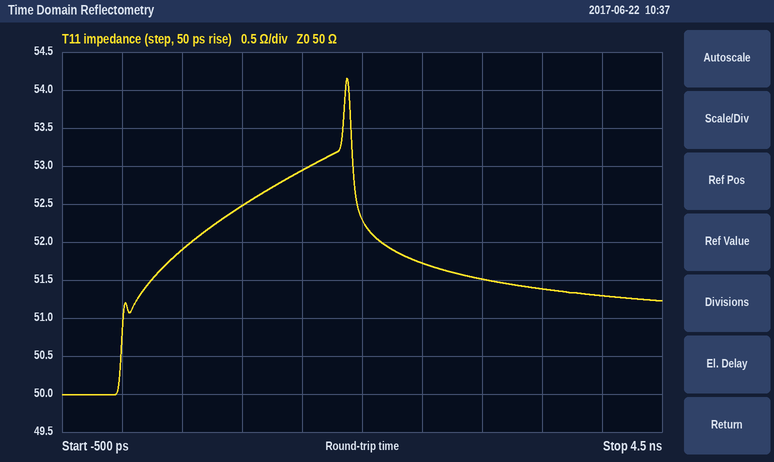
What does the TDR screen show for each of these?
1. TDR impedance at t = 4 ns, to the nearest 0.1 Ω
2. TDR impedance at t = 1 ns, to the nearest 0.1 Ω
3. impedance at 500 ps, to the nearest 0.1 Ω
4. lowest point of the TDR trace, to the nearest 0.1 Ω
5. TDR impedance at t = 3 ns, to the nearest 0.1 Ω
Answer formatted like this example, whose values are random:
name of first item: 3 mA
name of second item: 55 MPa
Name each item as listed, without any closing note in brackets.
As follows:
TDR impedance at t = 4 ns, to the nearest 0.1 Ω: 51.3 Ω
TDR impedance at t = 1 ns, to the nearest 0.1 Ω: 52.5 Ω
impedance at 500 ps, to the nearest 0.1 Ω: 51.9 Ω
lowest point of the TDR trace, to the nearest 0.1 Ω: 50.0 Ω
TDR impedance at t = 3 ns, to the nearest 0.1 Ω: 51.5 Ω
